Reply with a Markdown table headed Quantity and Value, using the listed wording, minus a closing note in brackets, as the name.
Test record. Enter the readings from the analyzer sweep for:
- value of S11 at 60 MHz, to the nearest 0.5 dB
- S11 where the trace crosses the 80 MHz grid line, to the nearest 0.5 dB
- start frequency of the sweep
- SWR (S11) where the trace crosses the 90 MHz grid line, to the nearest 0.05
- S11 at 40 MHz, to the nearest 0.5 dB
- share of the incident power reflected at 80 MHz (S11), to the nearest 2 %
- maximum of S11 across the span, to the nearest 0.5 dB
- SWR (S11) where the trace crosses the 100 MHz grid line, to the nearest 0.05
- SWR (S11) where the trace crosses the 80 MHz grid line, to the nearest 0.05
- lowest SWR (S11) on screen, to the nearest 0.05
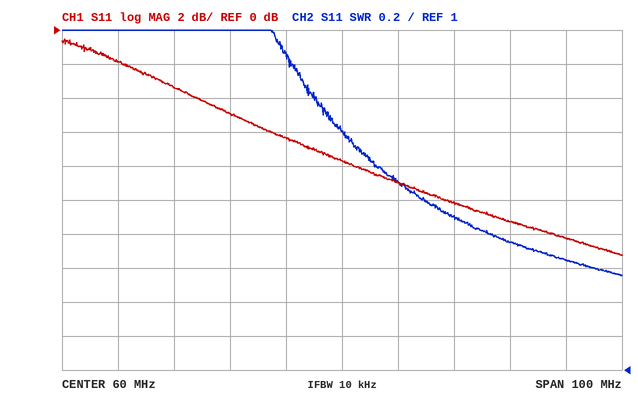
| Quantity | Value |
|---|---|
| value of S11 at 60 MHz, to the nearest 0.5 dB | -7.5 dB |
| S11 where the trace crosses the 80 MHz grid line, to the nearest 0.5 dB | -10.0 dB |
| start frequency of the sweep | 10 MHz |
| SWR (S11) where the trace crosses the 90 MHz grid line, to the nearest 0.05 | 1.75 |
| S11 at 40 MHz, to the nearest 0.5 dB | -5.0 dB |
| share of the incident power reflected at 80 MHz (S11), to the nearest 2 % | 10 % |
| maximum of S11 across the span, to the nearest 0.5 dB | -0.5 dB |
| SWR (S11) where the trace crosses the 100 MHz grid line, to the nearest 0.05 | 1.65 |
| SWR (S11) where the trace crosses the 80 MHz grid line, to the nearest 0.05 | 1.90 |
| lowest SWR (S11) on screen, to the nearest 0.05 | 1.55 |
